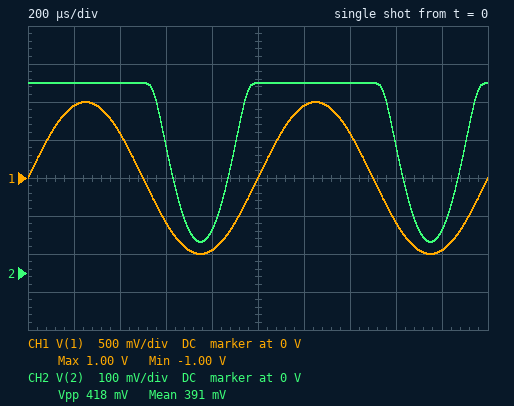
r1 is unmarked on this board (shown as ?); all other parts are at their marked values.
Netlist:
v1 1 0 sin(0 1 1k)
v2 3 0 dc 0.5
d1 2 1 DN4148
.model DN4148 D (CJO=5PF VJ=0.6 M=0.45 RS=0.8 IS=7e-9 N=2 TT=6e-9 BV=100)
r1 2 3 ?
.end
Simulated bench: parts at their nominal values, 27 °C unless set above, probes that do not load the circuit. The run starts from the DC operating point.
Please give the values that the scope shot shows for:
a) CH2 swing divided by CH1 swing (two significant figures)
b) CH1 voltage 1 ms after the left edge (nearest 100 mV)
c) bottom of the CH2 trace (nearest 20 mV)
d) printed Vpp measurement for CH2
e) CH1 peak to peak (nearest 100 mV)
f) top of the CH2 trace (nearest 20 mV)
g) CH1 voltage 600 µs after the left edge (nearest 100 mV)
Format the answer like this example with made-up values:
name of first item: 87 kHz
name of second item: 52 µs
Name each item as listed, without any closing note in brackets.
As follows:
CH2 swing divided by CH1 swing: 0.21
CH1 voltage 1 ms after the left edge: 0 V
bottom of the CH2 trace: 80 mV
printed Vpp measurement for CH2: 418 mV
CH1 peak to peak: 2.0 V
top of the CH2 trace: 500 mV
CH1 voltage 600 µs after the left edge: -600 mV
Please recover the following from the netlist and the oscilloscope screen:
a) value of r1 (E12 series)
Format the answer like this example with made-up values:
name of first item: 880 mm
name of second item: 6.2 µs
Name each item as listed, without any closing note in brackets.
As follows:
value of r1: 1.8 Ω
